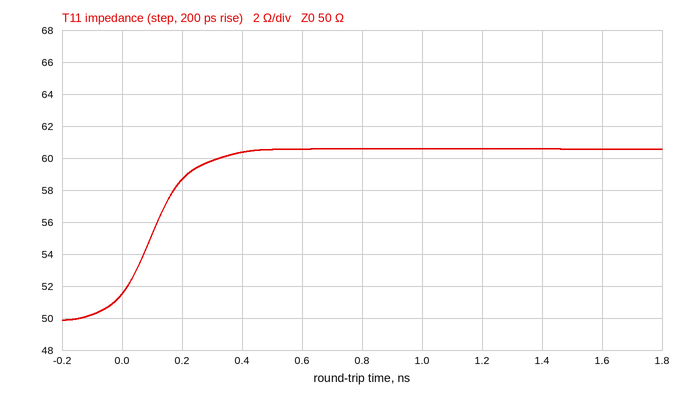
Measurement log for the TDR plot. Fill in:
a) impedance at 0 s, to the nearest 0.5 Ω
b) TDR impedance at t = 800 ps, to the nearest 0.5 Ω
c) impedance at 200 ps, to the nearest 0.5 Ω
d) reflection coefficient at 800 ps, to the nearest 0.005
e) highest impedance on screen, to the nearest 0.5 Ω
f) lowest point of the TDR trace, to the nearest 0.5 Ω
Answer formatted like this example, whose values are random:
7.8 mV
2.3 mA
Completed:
51.5 Ω
60.5 Ω
58.5 Ω
+0.095
60.5 Ω
50.0 Ω
